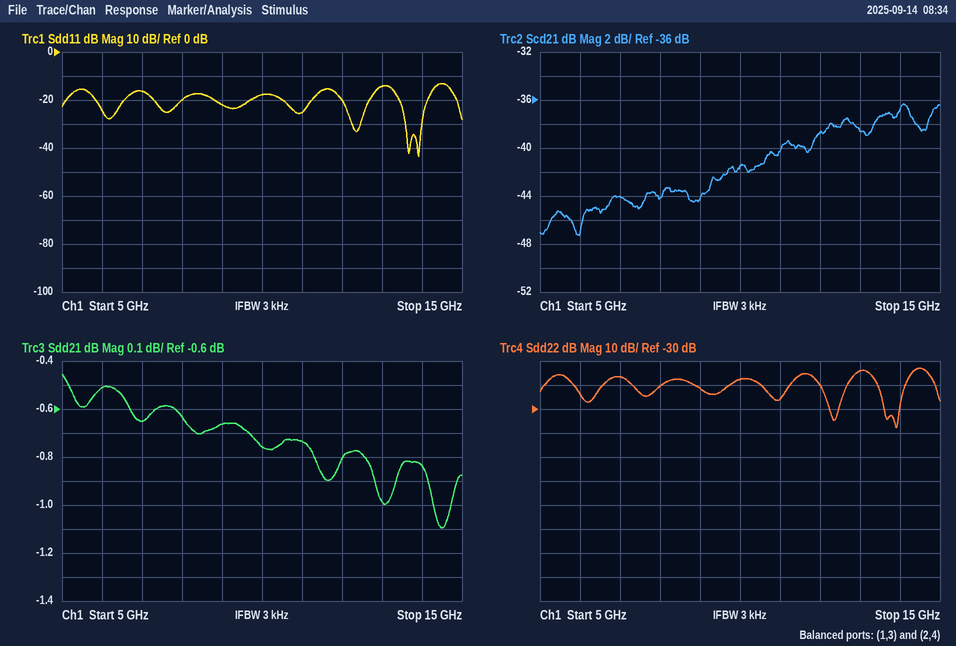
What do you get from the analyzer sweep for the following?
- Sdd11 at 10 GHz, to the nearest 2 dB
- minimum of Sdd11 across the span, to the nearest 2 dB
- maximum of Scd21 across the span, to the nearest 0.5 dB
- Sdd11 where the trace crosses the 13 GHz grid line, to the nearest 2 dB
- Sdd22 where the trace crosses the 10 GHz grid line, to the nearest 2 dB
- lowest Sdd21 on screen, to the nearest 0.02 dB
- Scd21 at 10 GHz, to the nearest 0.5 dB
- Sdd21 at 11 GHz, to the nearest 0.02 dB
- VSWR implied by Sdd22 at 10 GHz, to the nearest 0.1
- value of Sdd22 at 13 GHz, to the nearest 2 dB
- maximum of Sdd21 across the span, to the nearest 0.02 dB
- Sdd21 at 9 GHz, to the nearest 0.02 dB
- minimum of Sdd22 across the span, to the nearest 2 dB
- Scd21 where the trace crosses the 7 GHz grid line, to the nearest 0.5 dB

-18 dB
-44 dB
-36.5 dB
-14 dB
-18 dB
-1.10 dB
-41.5 dB
-0.74 dB
1.3
-14 dB
-0.46 dB
-0.66 dB
-38 dB
-44.0 dB
